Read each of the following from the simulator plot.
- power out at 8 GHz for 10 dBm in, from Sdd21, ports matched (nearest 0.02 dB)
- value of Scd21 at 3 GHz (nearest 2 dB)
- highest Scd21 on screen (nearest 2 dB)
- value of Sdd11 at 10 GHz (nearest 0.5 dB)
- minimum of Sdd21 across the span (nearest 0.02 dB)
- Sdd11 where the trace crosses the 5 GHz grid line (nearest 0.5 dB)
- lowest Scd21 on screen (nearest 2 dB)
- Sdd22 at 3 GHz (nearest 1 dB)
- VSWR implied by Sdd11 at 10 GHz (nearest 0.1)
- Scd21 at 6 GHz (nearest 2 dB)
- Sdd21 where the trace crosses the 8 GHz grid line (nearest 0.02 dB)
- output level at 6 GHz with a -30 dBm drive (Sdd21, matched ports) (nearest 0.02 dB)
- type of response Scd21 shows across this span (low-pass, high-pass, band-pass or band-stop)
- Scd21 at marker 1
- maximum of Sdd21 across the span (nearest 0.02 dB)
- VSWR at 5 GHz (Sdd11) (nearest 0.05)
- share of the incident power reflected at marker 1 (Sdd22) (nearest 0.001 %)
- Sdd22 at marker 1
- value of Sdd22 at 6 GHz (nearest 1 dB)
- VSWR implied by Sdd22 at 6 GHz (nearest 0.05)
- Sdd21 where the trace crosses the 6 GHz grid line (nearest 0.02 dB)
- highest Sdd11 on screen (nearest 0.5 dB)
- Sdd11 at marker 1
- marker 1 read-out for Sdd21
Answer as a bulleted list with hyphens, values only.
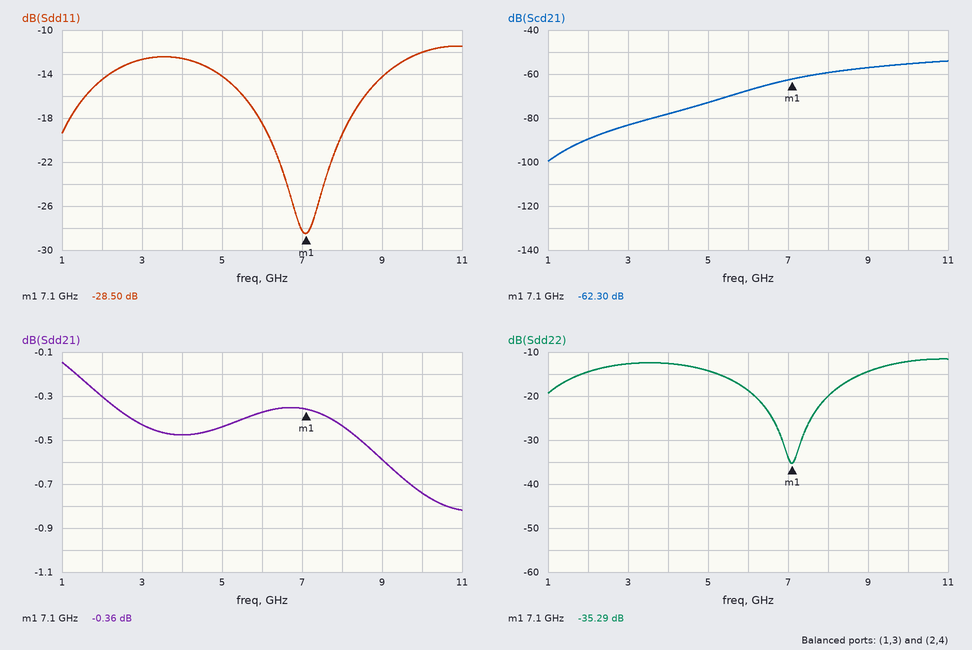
- 9.56 dBm
- -84 dB
- -54 dB
- -12.0 dB
- -0.82 dB
- -14.0 dB
- -100 dB
- -13 dB
- 1.7
- -68 dB
- -0.44 dB
- -30.38 dBm
- high-pass
- -62.30 dB
- -0.14 dB
- 1.50
- 0.030 %
- -35.29 dB
- -19 dB
- 1.25
- -0.38 dB
- -11.5 dB
- -28.50 dB
- -0.36 dB
